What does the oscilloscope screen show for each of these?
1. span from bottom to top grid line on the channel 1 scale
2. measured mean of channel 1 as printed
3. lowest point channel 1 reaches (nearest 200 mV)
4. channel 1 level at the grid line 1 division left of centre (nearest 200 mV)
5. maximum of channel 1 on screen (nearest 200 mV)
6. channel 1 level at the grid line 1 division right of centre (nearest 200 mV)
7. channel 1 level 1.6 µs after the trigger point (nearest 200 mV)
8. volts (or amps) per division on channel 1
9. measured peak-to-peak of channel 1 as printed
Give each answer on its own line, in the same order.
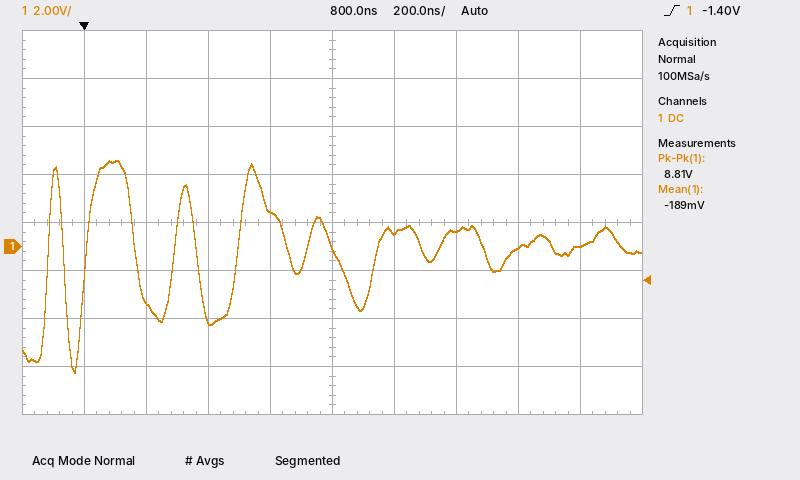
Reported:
16 V
-189 mV
-5.2 V
1.4 V
3.6 V
600 mV
0.0 V
2 V
8.81 V
